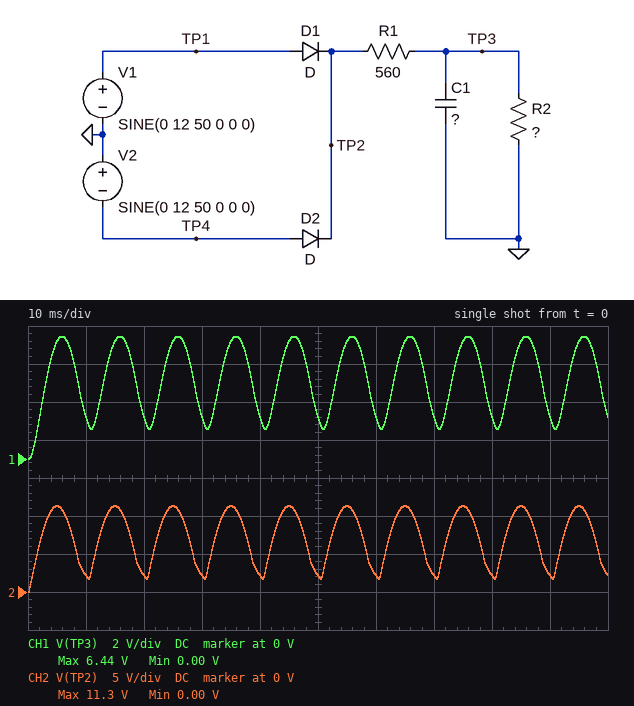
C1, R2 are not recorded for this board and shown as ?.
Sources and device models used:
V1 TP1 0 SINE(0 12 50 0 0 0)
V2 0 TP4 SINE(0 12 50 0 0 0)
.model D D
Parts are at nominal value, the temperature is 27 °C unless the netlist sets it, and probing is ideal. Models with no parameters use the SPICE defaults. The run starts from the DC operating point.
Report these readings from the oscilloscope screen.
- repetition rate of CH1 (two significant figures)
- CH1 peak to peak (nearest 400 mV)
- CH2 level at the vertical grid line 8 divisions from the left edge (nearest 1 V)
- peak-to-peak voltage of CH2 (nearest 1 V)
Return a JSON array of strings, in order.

["100 Hz", "6.4 V", "2 V", "11 V"]
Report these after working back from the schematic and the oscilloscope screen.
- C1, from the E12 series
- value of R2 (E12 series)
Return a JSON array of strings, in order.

["2.7 µF", "820 Ω"]
